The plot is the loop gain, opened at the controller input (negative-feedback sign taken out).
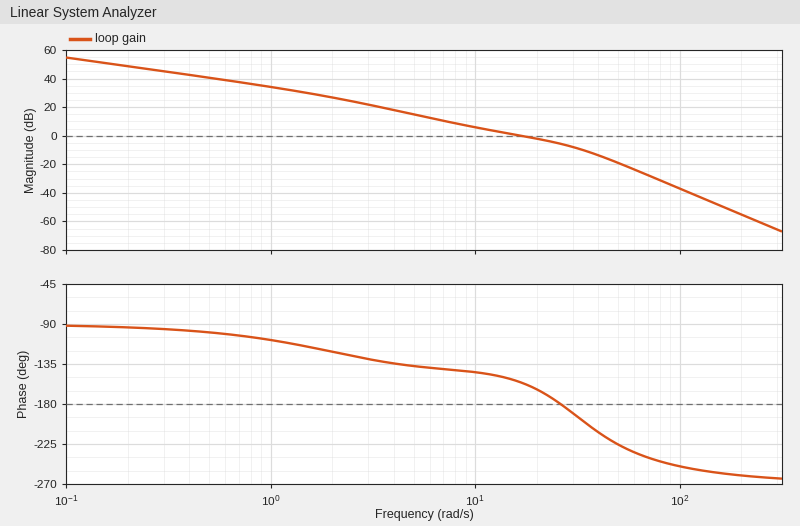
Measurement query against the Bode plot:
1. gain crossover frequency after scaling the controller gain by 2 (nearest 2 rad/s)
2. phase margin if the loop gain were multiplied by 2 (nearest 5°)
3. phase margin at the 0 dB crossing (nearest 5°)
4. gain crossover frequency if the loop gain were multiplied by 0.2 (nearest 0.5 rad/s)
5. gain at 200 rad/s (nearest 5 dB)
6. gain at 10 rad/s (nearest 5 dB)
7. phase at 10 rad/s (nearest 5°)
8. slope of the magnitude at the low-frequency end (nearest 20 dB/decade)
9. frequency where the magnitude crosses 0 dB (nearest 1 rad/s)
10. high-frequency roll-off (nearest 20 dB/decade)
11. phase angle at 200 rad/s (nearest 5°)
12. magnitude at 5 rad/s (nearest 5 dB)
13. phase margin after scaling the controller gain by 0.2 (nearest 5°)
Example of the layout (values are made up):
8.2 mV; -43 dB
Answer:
26 rad/s; 0°; 25°; 5.5 rad/s; -55 dB; 5 dB; -145°; -20 dB/decade; 17 rad/s; -60 dB/decade; -260°; 15 dB; 40°
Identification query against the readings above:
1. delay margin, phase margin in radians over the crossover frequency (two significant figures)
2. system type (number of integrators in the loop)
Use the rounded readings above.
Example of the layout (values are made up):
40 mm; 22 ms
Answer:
0.026 s; 1
